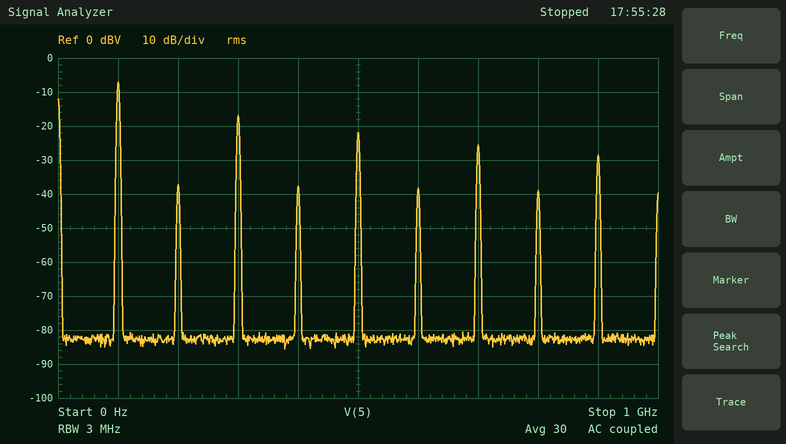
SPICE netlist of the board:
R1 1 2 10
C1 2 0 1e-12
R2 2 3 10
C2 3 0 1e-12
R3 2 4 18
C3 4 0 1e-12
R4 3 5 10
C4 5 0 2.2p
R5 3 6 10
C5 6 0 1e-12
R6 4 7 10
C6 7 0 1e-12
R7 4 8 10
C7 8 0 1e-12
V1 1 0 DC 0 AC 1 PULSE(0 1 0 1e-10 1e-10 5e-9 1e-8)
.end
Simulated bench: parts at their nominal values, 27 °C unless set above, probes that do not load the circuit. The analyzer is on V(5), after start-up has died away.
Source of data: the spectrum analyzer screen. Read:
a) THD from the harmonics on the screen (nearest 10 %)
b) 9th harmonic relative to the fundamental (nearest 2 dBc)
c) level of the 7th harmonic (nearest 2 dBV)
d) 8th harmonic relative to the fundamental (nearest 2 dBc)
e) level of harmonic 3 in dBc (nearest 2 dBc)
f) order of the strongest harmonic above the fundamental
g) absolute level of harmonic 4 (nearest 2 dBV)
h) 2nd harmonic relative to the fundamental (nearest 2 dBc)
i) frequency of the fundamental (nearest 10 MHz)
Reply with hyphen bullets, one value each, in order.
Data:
- 40 %
- -22 dBc
- -26 dBV
- -32 dBc
- -10 dBc
- 3
- -38 dBV
- -30 dBc
- 100 MHz
